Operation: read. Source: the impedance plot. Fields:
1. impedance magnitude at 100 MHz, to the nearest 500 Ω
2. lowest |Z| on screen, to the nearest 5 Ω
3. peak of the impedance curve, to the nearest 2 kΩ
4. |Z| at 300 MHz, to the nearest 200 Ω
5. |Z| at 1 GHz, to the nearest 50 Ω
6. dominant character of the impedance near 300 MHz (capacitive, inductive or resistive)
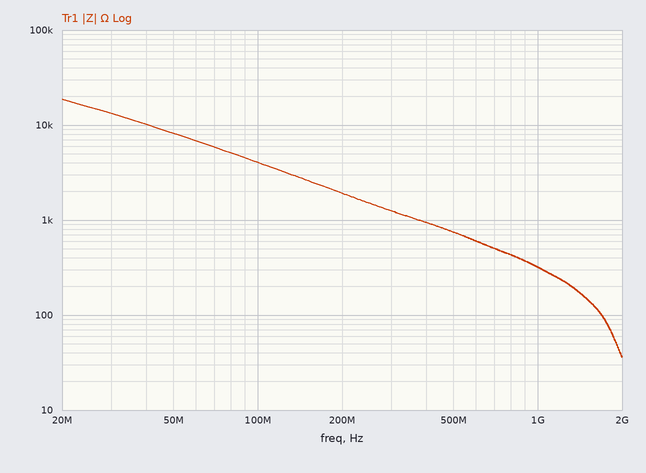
4.0 kΩ
35 Ω
18 kΩ
1.2 kΩ
300 Ω
capacitive
